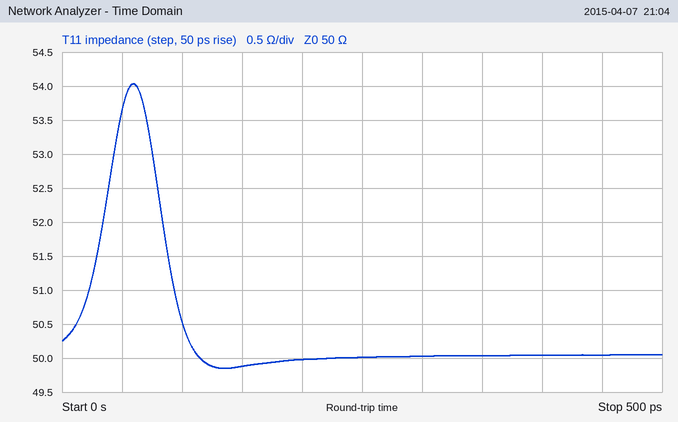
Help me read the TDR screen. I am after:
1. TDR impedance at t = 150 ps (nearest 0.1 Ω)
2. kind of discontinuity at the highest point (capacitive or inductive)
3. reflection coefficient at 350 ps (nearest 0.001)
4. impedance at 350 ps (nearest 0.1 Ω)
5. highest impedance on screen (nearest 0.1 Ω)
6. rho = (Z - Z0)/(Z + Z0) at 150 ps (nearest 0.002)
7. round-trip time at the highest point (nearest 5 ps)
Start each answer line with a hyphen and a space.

- 49.9 Ω
- inductive
- 0.000
- 50.0 Ω
- 54.0 Ω
- -0.002
- 60 ps
